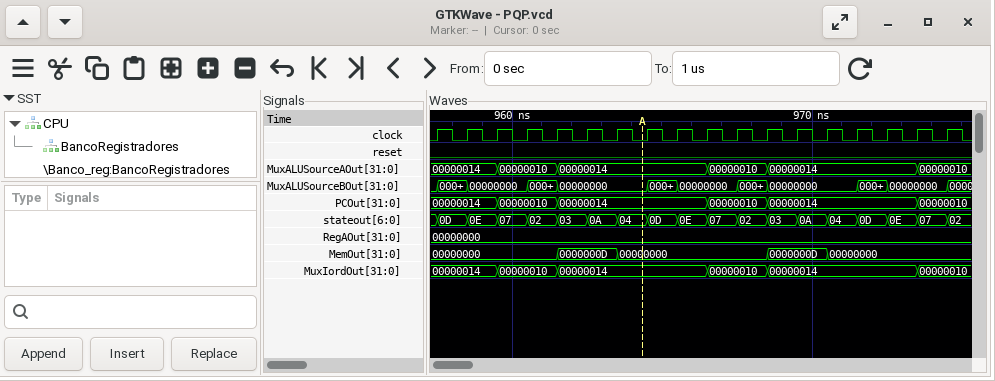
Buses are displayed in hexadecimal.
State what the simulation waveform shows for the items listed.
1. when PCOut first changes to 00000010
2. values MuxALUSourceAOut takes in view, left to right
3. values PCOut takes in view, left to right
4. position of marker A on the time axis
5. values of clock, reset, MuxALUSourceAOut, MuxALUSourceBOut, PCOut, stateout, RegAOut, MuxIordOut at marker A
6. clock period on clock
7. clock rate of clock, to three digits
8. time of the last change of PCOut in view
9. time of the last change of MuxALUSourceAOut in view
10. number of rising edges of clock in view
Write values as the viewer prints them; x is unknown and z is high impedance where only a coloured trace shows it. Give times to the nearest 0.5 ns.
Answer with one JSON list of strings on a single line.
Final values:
["959.5 ns", "00000014, 00000010, 00000014, 00000010, 00000014, 00000010", "00000014, 00000010, 00000014, 00000010, 00000014, 00000010", "964.5 ns", "clock=0, reset=0, MuxALUSourceAOut=00000014, MuxALUSourceBOut=00000000, PCOut=00000014, stateout=04, RegAOut=00000000, MuxIordOut=00000014", "1 ns", "1.00 GHz", "973.5 ns", "973.5 ns", "18"]
